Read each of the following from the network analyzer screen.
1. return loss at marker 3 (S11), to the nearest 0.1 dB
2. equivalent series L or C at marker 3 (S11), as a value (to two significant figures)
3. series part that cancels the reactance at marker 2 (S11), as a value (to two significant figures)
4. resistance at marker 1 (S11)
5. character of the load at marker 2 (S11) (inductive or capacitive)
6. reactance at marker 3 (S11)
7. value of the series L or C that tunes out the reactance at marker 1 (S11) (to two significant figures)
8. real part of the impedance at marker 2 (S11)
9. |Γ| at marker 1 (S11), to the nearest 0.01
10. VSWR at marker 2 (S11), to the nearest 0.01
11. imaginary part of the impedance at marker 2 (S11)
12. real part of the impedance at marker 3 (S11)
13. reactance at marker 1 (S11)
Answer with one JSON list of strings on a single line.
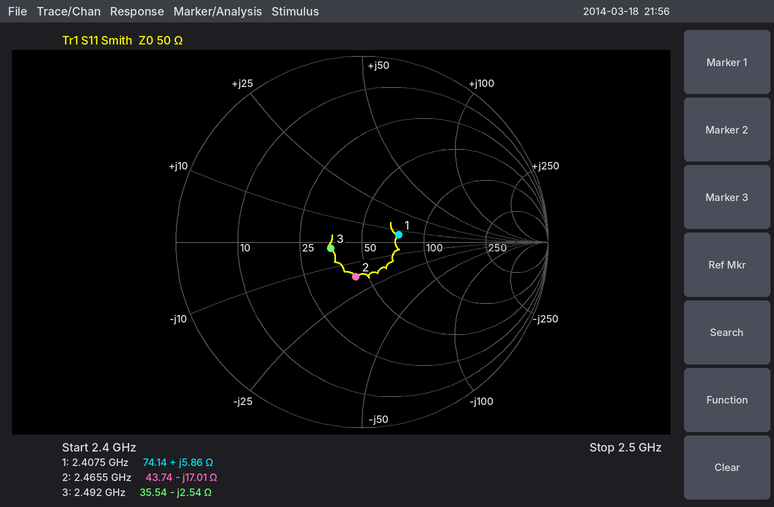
["15.3 dB", "25 pF", "1.1 nH", "74.14 Ω", "capacitive", "-2.54 Ω", "11 pF", "43.74 Ω", "0.20", "1.47", "-17.01 Ω", "35.54 Ω", "+5.86 Ω"]
